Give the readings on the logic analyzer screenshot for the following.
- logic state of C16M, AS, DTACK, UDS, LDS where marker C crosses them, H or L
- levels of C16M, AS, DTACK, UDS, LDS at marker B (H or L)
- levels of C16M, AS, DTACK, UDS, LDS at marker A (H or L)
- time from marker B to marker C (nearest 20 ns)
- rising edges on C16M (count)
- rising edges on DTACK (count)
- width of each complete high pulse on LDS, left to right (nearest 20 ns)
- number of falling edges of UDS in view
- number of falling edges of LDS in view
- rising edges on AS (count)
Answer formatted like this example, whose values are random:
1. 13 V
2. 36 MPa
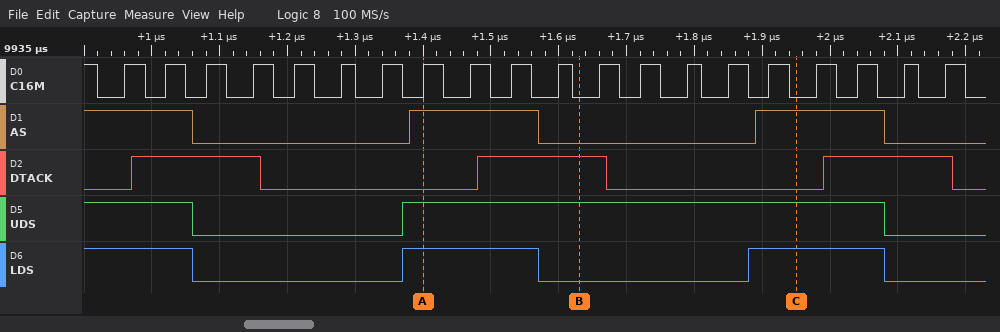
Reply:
1. C16M=L, AS=H, DTACK=L, UDS=H, LDS=H
2. C16M=L, AS=L, DTACK=H, UDS=H, LDS=L
3. C16M=H, AS=H, DTACK=L, UDS=H, LDS=H
4. 320 ns
5. 20
6. 3
7. 200 ns, 200 ns
8. 2
9. 3
10. 2
